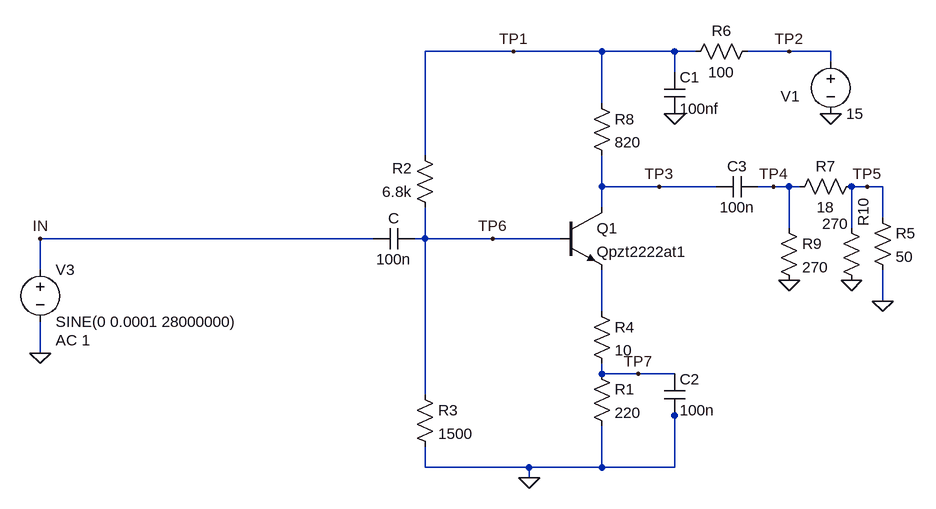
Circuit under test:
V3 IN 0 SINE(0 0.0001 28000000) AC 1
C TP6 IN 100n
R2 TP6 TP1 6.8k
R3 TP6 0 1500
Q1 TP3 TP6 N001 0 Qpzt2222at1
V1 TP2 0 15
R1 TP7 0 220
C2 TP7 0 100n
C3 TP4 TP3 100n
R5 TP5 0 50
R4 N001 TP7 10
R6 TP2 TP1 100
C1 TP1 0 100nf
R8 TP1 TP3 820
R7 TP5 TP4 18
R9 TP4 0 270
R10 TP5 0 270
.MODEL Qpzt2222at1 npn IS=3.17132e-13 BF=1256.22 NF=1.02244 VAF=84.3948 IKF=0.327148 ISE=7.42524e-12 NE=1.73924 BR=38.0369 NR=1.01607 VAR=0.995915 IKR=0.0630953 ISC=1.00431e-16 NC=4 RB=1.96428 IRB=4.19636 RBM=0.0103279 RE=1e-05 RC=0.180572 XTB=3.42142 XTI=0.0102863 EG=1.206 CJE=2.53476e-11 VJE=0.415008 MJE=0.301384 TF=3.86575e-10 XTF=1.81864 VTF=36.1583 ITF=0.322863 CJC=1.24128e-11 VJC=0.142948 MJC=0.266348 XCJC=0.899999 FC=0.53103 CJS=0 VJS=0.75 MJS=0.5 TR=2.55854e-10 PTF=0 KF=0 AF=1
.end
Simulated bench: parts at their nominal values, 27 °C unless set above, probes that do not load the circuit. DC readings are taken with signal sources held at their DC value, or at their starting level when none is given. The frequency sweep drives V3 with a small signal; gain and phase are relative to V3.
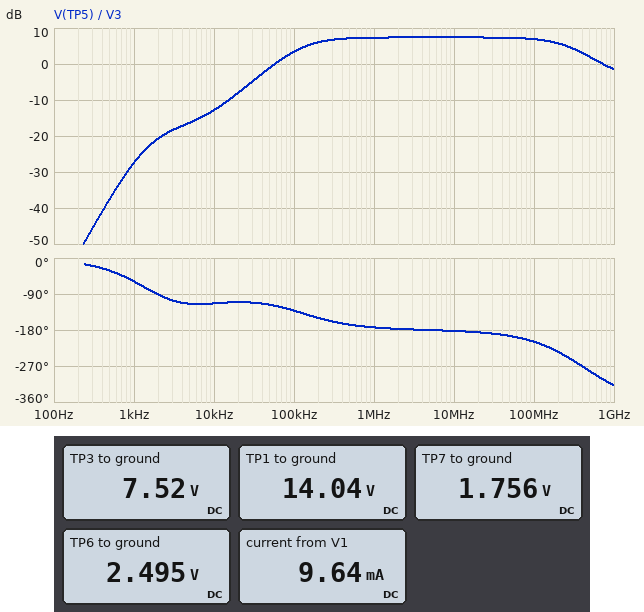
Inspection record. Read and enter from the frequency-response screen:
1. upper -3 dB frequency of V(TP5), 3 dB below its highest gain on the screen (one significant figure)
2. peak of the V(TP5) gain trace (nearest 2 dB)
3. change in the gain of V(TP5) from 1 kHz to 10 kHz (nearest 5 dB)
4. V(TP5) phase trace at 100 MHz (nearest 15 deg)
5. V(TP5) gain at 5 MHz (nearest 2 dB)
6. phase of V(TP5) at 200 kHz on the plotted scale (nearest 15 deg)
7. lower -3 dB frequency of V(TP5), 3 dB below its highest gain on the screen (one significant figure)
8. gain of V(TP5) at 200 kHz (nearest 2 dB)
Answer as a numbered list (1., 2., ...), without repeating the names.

1. 300 MHz
2. 8 dB
3. 15 dB
4. -210 deg
5. 8 dB
6. -150 deg
7. 100 kHz
8. 6 dB
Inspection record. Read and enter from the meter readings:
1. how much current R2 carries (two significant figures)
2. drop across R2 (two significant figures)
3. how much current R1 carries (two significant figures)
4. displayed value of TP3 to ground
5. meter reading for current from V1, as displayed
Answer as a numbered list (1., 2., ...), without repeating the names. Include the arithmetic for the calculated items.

1. (14.04 V - 2.495 V) / 6.8 kΩ = 1.7 mA
2. 14.04 V - 2.495 V = 12 V
3. (1.756 V) / 220 Ω = 8.0 mA
4. 7.52 V
5. 9.64 mA
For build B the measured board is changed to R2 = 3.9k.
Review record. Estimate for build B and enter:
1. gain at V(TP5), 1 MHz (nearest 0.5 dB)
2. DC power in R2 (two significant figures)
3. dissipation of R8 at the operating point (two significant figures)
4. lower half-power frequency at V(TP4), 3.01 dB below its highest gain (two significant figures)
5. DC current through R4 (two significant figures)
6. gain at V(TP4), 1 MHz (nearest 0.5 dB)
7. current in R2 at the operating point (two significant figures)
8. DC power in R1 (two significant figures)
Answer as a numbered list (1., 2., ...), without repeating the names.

1. 5.5 dB
2. 25 mW
3. 130 mW
4. 120 kHz
5. 13 mA
6. 8.5 dB
7. 2.5 mA
8. 36 mW
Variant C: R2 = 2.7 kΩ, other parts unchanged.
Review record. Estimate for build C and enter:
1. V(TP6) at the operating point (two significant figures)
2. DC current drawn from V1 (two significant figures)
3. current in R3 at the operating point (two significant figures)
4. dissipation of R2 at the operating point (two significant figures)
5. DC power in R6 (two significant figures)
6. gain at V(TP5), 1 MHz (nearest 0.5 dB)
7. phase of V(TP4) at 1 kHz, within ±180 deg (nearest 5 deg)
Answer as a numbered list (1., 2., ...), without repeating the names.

1. 3.8 V
2. 16 mA
3. 2.5 mA
4. 34 mW
5. 26 mW
6. -26.0 dB
7. 160 deg
